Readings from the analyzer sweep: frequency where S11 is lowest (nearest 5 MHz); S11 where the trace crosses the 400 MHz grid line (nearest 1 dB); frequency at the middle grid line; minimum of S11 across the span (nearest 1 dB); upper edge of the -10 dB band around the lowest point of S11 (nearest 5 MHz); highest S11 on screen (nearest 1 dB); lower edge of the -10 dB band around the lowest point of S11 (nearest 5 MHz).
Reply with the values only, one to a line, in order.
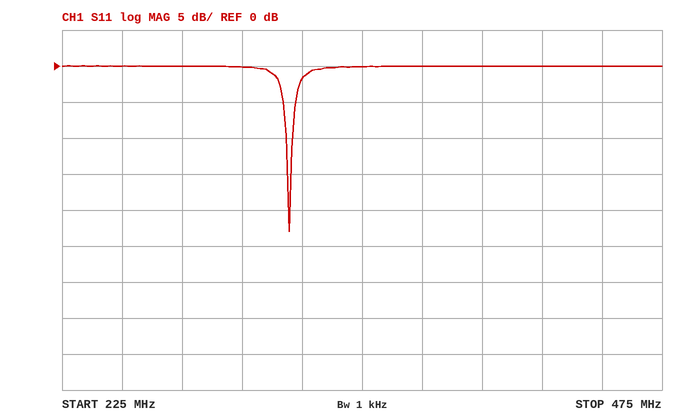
320 MHz
0 dB
350 MHz
-23 dB
320 MHz
0 dB
320 MHz
